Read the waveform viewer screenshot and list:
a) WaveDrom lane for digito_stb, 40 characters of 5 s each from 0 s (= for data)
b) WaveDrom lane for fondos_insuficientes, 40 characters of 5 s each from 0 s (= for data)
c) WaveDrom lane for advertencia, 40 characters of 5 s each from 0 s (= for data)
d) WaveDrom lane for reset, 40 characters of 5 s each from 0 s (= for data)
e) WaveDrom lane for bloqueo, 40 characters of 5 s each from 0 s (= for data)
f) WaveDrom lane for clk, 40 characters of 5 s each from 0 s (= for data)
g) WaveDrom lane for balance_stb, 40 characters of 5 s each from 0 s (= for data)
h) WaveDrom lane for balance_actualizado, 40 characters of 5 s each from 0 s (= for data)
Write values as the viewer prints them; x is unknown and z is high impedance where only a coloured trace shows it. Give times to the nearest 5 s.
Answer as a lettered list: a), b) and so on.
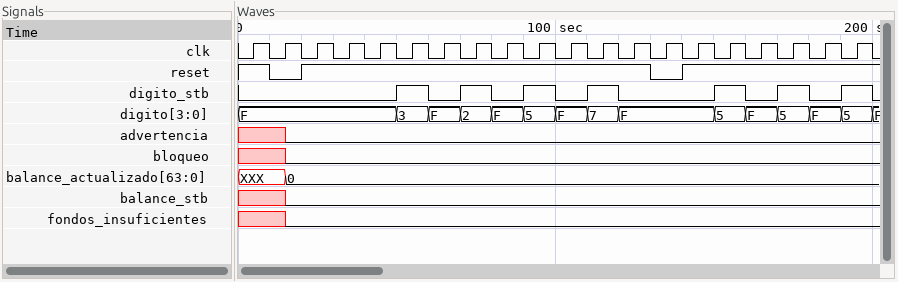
a) {name: 'digito_stb', wave: '0.........1.0.1.0.1.0.1.0.....1.0.1.0.1.'}
b) {name: 'fondos_insuficientes', wave: 'x..0....................................'}
c) {name: 'advertencia', wave: 'x..0....................................'}
d) {name: 'reset', wave: '1.0.1.....................0.1...........'}
e) {name: 'bloqueo', wave: 'x..0....................................'}
f) {name: 'clk', wave: '0101010101010101010101010101010101010101'}
g) {name: 'balance_stb', wave: 'x..0....................................'}
h) {name: 'balance_actualizado', wave: 'x..=....................................', data: '0'}
